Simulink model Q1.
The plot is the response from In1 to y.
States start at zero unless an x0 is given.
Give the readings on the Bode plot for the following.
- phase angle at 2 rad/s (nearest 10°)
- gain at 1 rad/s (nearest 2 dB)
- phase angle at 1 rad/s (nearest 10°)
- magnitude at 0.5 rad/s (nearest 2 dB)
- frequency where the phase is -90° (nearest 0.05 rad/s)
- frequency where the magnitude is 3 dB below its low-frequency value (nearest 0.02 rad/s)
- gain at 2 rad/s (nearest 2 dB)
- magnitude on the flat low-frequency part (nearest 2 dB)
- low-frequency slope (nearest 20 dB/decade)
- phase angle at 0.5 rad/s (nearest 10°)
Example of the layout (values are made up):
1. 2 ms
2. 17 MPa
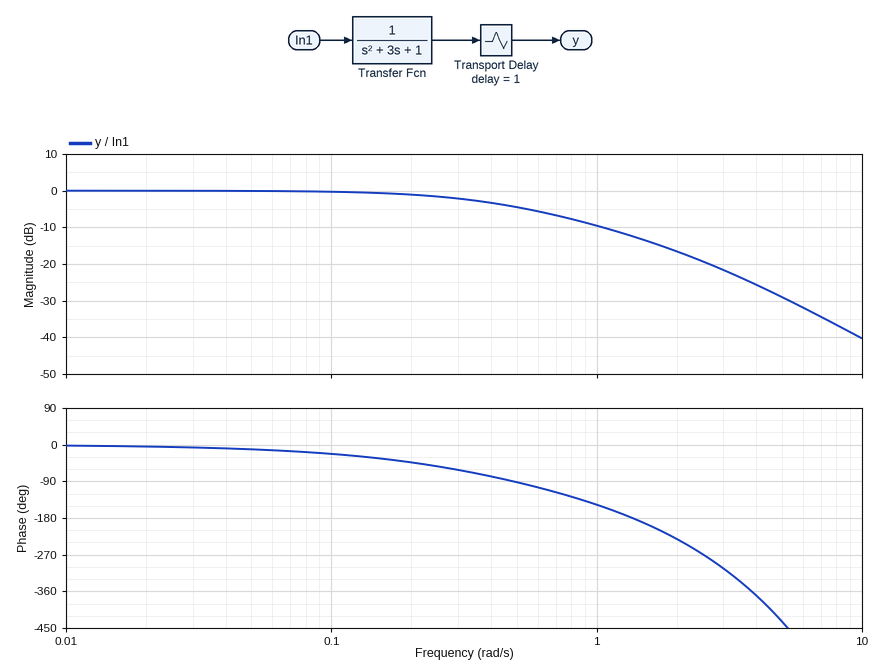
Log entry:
1. -230°
2. -10 dB
3. -150°
4. -4 dB
5. 0.50 rad/s
6. 0.38 rad/s
7. -16 dB
8. 0 dB
9. 0 dB/decade
10. -90°
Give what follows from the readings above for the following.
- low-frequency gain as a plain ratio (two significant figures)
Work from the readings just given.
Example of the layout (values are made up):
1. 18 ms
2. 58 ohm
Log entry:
1. 1.0
